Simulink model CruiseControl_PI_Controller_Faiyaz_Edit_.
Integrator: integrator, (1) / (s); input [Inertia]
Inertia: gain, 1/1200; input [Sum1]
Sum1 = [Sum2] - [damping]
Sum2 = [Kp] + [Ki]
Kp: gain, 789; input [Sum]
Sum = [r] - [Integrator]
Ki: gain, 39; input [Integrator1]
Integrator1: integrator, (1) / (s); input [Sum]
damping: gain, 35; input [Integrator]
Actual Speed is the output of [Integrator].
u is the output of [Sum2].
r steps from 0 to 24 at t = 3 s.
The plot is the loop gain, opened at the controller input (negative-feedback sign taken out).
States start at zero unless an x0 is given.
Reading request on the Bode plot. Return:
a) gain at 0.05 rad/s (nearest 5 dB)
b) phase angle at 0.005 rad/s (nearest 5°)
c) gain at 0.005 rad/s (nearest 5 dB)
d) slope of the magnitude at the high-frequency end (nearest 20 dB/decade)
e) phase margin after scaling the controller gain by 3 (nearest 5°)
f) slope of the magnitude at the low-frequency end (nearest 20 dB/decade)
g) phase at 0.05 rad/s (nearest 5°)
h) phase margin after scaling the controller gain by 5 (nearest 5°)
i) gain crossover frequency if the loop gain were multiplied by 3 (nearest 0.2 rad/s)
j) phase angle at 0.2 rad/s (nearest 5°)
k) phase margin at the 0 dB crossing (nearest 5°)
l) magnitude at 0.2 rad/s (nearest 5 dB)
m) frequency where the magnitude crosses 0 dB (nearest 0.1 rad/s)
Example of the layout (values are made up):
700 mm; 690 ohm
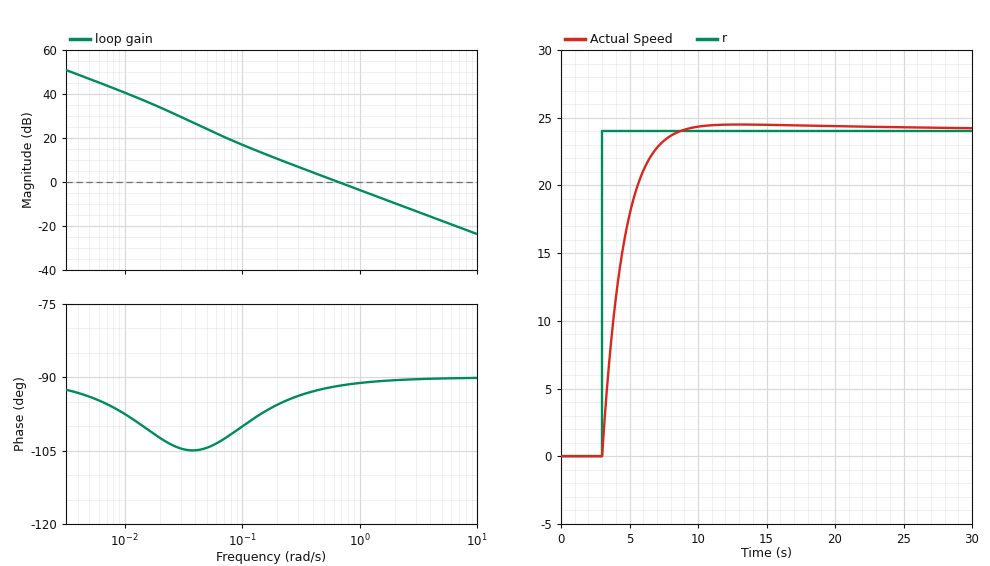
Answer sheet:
25 dB; -95°; 45 dB; -20 dB/decade; 90°; -20 dB/decade; -105°; 90°; 2.0 rad/s; -95°; 90°; 10 dB; 0.7 rad/s
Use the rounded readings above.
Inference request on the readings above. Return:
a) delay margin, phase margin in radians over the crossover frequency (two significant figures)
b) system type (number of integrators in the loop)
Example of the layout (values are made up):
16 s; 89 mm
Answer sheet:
2.2 s; 1
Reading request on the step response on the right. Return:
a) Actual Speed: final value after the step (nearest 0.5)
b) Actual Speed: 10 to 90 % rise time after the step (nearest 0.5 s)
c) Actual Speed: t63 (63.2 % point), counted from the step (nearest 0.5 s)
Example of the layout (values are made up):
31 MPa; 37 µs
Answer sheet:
24.0; 3.0 s; 1.5 s
